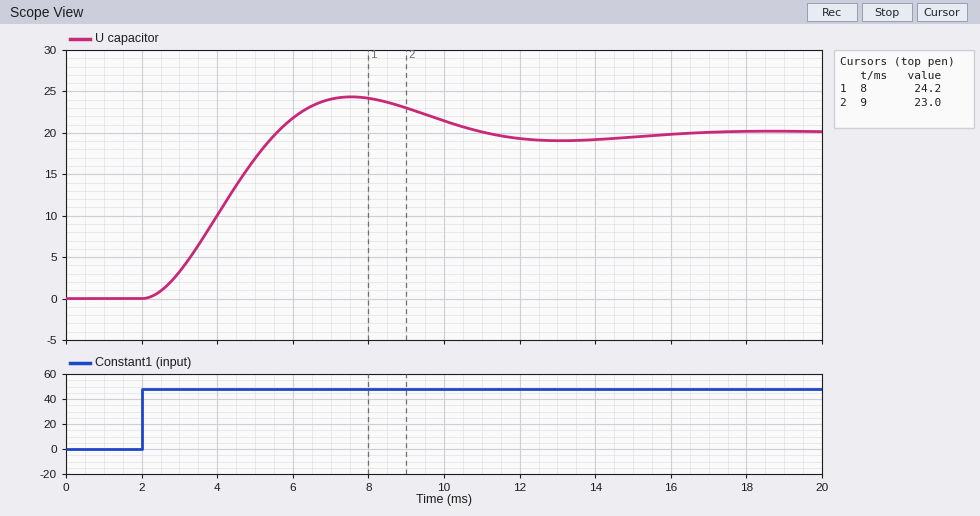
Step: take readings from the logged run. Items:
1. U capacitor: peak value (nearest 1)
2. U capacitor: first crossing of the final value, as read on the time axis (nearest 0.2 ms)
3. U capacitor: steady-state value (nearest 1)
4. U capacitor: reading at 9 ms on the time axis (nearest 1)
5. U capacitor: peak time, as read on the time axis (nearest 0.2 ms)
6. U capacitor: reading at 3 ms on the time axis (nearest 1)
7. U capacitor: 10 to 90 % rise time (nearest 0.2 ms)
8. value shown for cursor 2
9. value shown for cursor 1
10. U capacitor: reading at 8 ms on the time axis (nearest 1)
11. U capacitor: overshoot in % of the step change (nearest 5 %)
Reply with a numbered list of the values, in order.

1. 24
2. 5.6 ms
3. 20
4. 23
5. 7.6 ms
6. 3
7. 2.4 ms
8. 23.0
9. 24.2
10. 24
11. 20 %
